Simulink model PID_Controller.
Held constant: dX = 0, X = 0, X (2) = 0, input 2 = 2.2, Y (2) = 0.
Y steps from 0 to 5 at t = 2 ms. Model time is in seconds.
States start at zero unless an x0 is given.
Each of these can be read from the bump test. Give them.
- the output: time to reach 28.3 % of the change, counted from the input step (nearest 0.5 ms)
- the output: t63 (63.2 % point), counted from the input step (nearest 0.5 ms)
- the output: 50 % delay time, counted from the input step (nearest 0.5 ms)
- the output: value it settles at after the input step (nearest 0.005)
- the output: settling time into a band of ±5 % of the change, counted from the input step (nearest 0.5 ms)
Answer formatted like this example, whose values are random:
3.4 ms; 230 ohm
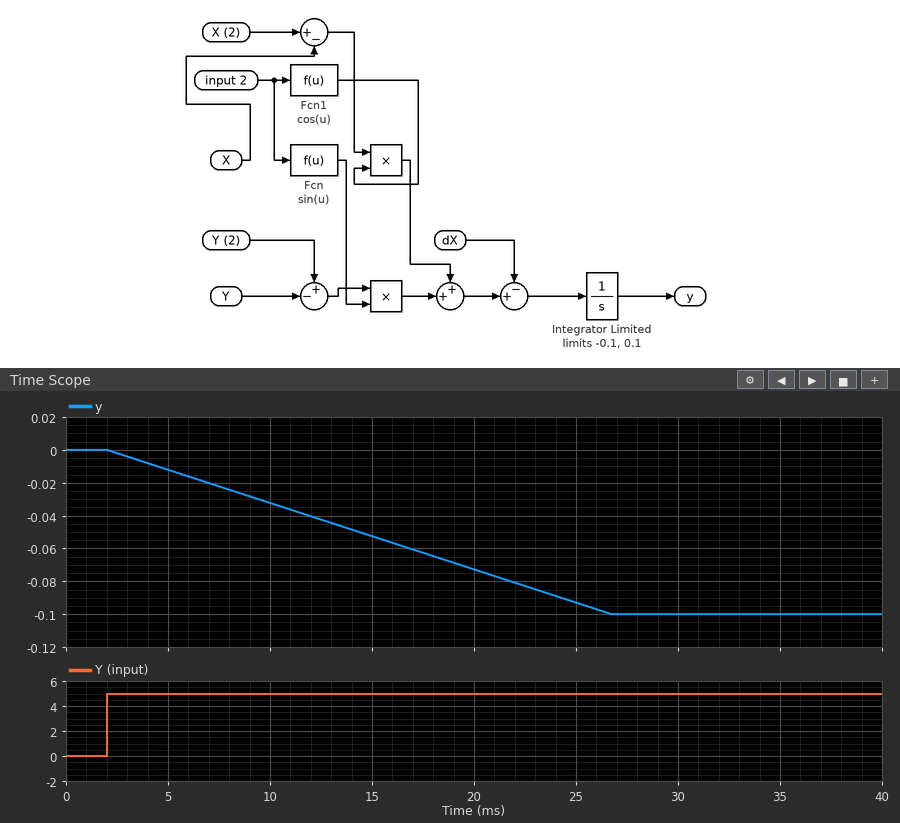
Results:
7.0 ms; 15.5 ms; 12.5 ms; -0.100; 23.5 ms
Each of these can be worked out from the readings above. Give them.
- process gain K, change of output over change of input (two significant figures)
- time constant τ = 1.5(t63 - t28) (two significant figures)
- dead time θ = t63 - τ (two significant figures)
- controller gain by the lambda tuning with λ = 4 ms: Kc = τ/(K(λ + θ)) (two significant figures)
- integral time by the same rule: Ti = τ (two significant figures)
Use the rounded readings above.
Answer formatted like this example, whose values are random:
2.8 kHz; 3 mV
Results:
-0.020; 13 ms; 2.5 ms; -100; 13 ms
